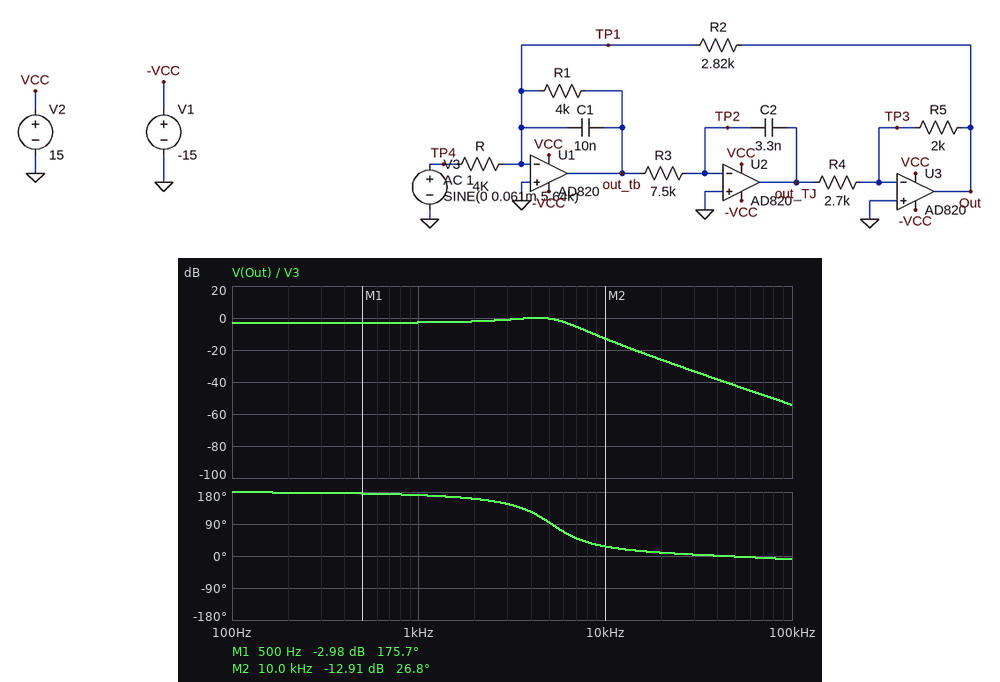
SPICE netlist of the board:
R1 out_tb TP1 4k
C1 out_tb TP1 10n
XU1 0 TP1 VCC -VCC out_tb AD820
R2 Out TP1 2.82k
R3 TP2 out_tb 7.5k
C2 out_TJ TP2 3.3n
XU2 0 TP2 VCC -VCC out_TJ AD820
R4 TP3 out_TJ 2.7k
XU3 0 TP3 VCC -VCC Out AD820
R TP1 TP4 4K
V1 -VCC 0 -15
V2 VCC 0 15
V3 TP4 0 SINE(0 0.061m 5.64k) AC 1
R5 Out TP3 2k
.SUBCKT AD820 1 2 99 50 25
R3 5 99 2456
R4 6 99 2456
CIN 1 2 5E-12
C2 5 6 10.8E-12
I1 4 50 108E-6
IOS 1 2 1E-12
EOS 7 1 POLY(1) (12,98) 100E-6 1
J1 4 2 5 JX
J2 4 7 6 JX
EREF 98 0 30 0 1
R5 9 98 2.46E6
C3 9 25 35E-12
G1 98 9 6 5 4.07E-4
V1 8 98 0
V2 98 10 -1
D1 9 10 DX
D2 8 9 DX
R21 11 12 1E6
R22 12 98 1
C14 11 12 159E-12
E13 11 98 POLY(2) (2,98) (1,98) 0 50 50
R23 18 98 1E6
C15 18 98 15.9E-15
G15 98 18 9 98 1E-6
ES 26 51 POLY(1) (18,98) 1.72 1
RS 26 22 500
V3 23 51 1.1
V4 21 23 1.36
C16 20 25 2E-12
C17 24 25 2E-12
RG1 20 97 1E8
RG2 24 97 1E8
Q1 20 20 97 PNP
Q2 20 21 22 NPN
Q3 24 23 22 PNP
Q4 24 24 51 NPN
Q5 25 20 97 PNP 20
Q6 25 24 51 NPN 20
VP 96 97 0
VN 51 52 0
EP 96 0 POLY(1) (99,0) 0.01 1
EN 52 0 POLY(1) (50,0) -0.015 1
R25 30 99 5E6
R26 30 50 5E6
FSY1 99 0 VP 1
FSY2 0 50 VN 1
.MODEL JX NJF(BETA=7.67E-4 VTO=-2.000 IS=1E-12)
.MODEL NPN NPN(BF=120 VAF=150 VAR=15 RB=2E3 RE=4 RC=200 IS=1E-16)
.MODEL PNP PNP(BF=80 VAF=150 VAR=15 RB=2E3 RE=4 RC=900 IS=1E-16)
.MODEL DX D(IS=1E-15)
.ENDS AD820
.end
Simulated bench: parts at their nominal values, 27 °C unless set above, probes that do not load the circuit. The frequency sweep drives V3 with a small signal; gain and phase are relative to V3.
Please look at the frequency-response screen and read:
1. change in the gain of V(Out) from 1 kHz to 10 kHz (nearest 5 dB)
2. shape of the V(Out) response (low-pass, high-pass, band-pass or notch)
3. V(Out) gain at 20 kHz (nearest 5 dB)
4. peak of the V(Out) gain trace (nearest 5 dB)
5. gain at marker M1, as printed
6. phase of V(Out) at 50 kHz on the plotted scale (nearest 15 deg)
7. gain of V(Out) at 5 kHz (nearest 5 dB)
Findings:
-10 dB
low-pass
-25 dB
0 dB
-2.98 dB
0 deg
0 dB
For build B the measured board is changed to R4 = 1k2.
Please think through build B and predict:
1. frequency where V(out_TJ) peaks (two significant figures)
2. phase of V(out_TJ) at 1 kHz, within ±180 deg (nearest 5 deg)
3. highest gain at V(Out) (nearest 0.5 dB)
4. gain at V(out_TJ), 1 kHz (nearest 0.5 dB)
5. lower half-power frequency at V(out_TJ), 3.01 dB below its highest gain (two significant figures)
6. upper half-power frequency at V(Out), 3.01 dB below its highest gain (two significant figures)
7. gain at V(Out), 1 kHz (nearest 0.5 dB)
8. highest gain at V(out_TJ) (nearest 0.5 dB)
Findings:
7.3 kHz
-5 deg
3.5 dB
-7.5 dB
4.9 kHz
9.0 kHz
-3.0 dB
-1.0 dB
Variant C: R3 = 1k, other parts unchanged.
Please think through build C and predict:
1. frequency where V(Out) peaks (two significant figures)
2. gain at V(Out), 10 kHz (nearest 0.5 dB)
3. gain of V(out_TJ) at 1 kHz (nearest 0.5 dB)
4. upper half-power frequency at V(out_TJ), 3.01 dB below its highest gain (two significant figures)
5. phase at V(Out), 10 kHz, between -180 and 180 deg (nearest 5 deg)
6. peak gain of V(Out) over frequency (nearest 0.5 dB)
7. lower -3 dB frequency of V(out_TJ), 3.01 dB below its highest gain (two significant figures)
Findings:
14 kHz
2.5 dB
-0.5 dB
15 kHz
160 deg
9.0 dB
12 kHz
